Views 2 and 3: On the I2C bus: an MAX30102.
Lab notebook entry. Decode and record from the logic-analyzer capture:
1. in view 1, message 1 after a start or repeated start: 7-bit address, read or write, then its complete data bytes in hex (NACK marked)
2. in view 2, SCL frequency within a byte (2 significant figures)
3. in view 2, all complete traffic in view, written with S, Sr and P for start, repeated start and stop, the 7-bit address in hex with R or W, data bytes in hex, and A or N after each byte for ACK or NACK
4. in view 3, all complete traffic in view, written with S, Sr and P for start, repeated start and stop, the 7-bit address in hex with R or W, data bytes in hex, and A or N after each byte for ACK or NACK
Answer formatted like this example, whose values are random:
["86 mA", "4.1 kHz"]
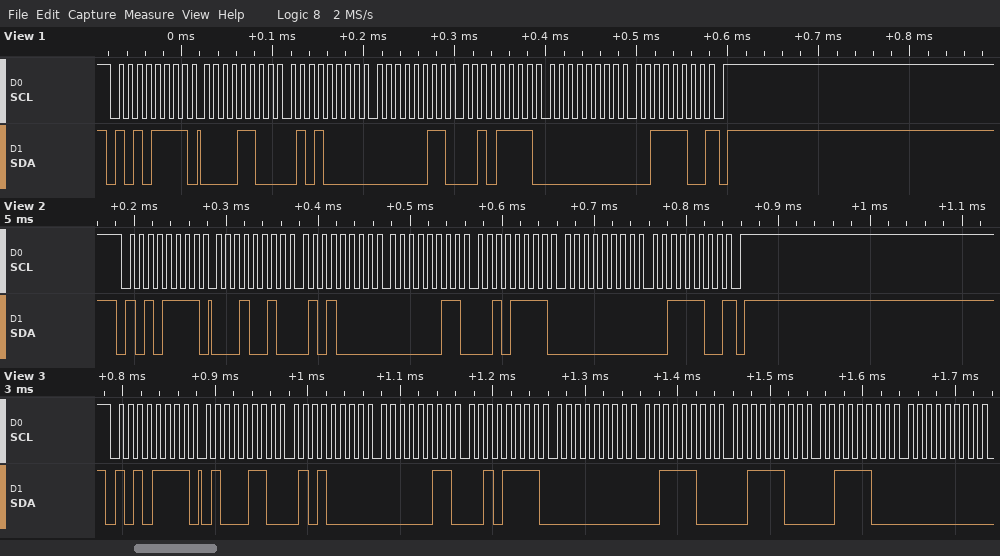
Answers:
["0x57 read: 0C 50 03 2F 00 3C NACK", "100 kHz", "S 57R A 12 A 50 A 03 A 2F A 00 A 3C N P", "S 57R A 46 A 50 A 03 A 2F A 00 A 3C A 3C A 3C A 00 A"]
